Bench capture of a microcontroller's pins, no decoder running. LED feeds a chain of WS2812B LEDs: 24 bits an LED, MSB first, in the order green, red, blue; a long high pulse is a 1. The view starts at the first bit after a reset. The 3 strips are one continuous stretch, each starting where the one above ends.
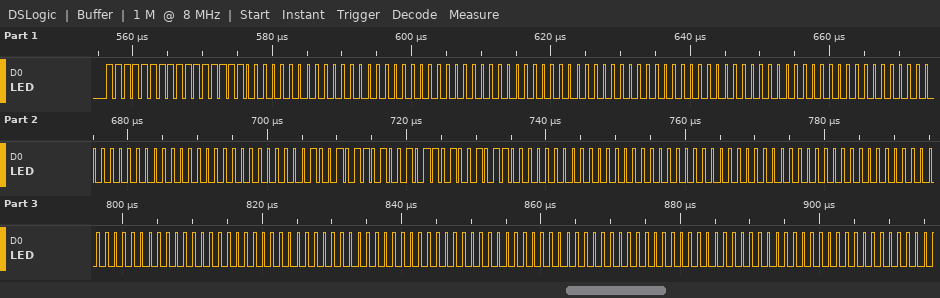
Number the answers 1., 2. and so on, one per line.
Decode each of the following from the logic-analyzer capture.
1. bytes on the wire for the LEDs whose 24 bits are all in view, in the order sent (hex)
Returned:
1. FF FF 00 00 00 00 00 00 00 00 00 00 00 00 00 96 96 96 00 00 00 00 00 00 00 00 00 00 00 00 00 00 00 00 00 00
